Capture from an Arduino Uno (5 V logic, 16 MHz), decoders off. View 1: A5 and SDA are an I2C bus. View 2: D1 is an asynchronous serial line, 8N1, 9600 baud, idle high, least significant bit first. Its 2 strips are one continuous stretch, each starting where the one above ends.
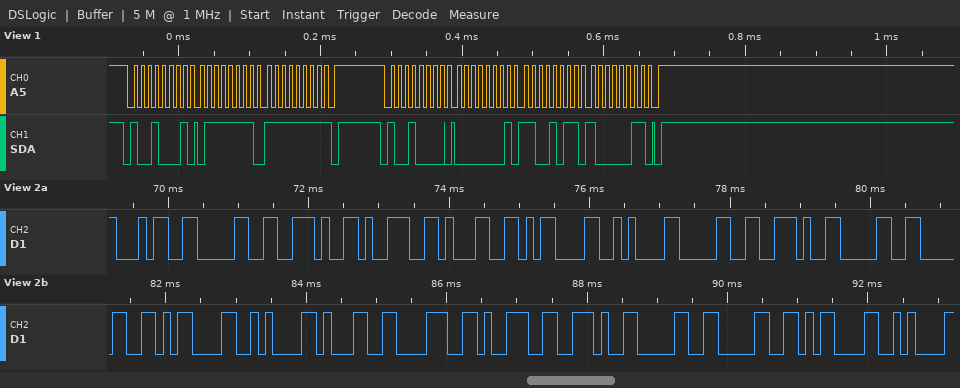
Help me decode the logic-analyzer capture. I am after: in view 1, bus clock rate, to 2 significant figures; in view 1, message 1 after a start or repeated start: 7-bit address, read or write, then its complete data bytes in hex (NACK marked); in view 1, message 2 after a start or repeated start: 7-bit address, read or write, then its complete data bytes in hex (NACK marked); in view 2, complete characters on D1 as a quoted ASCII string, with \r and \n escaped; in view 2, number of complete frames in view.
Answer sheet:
100 kHz
0x48 read: 7F FF NACK
0x48 write: 01 CB 83
"40.91\r\n0.00\r\n189.00\r\n"
21
